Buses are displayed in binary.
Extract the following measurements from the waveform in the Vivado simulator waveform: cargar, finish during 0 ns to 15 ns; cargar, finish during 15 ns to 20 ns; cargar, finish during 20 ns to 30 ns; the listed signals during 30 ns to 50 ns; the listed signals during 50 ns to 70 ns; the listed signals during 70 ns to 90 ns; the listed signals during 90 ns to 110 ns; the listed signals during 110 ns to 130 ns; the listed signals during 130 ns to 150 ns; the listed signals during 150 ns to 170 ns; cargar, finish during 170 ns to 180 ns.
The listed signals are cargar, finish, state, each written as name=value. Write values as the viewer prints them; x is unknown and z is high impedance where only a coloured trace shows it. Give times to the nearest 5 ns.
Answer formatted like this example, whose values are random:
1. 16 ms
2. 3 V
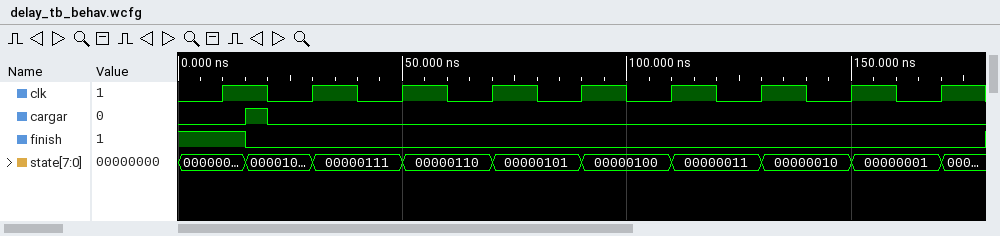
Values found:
1. cargar=0, finish=1
2. cargar=1, finish=0
3. cargar=0, finish=0
4. cargar=0, finish=0, state=00000111
5. cargar=0, finish=0, state=00000110
6. cargar=0, finish=0, state=00000101
7. cargar=0, finish=0, state=00000100
8. cargar=0, finish=0, state=00000011
9. cargar=0, finish=0, state=00000010
10. cargar=0, finish=0, state=00000001
11. cargar=0, finish=0
